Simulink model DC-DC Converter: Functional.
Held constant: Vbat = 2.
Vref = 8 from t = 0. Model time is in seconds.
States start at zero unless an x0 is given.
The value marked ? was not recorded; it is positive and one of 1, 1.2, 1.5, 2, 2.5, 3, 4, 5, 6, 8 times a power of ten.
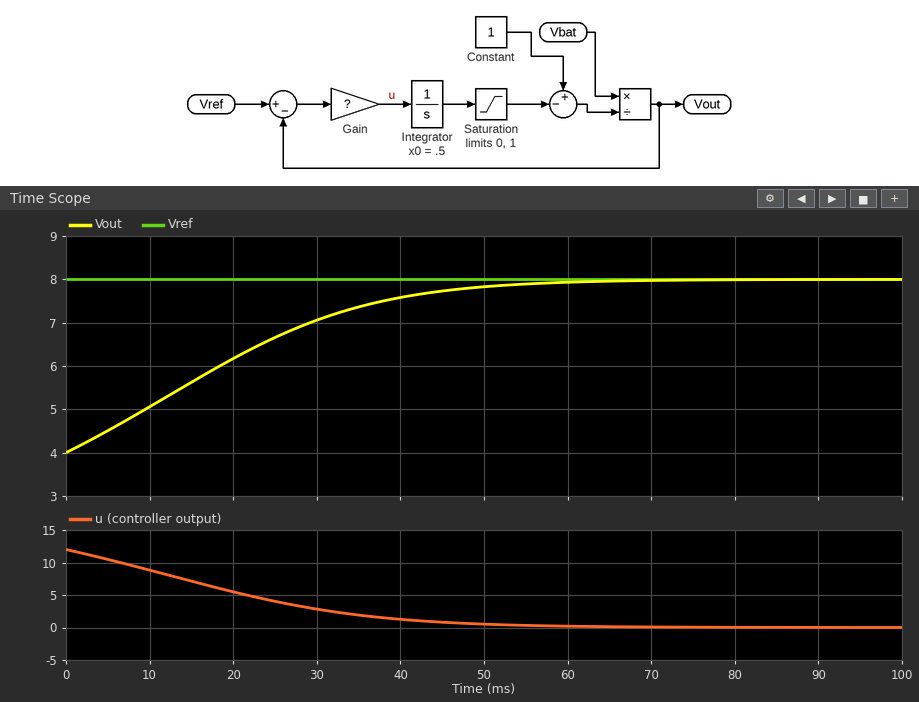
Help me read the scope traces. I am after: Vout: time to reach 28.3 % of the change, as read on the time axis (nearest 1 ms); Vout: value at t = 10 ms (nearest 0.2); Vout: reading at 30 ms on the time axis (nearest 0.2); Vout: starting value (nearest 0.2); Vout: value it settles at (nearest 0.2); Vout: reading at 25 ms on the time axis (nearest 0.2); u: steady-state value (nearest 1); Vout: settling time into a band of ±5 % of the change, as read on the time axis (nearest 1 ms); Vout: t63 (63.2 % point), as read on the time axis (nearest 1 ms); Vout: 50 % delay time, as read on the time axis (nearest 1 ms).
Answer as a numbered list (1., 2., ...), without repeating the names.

1. 11 ms
2. 5.0
3. 7.0
4. 4.0
5. 8.0
6. 6.6
7. 0
8. 48 ms
9. 24 ms
10. 18 ms
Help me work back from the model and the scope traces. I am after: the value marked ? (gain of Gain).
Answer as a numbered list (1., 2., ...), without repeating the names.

1. 3
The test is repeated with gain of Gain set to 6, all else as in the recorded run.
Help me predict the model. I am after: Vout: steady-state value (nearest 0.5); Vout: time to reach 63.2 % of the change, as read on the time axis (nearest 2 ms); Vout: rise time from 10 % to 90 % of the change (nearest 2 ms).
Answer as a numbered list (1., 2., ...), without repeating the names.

1. 8.0
2. 12 ms
3. 18 ms
